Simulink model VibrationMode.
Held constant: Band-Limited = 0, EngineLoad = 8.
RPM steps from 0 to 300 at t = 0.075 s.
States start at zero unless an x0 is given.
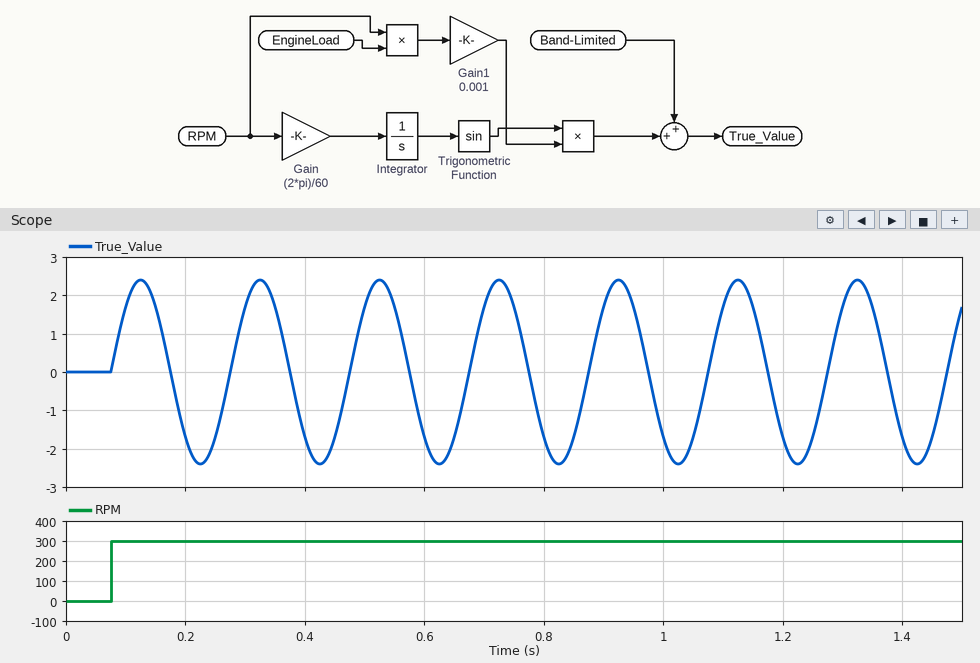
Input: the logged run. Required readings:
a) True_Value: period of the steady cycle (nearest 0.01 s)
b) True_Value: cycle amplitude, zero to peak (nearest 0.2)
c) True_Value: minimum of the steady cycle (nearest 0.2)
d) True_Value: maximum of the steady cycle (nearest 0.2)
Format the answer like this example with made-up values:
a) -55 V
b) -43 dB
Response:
a) 0.20 s
b) 2.4
c) -2.4
d) 2.4
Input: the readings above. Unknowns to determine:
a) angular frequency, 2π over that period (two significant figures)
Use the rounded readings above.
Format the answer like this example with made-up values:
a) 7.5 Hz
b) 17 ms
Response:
a) 31 rad/s
